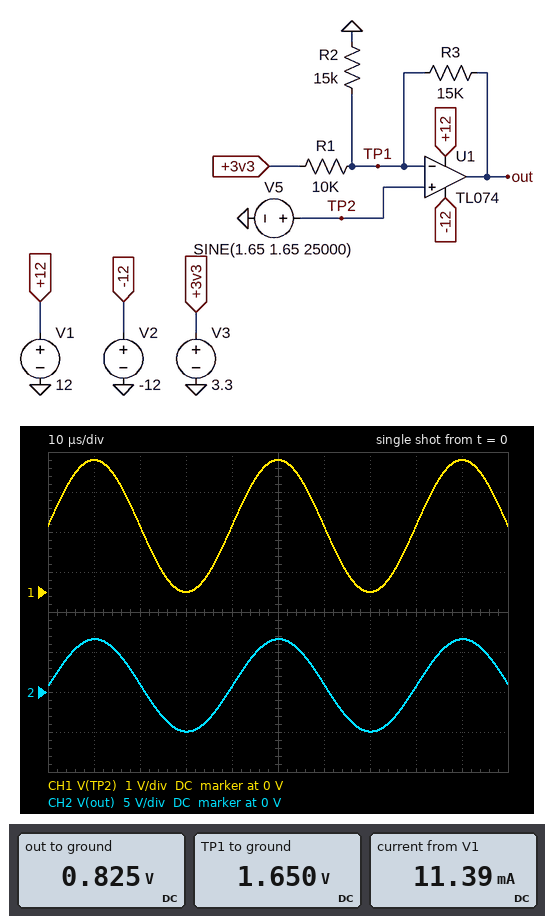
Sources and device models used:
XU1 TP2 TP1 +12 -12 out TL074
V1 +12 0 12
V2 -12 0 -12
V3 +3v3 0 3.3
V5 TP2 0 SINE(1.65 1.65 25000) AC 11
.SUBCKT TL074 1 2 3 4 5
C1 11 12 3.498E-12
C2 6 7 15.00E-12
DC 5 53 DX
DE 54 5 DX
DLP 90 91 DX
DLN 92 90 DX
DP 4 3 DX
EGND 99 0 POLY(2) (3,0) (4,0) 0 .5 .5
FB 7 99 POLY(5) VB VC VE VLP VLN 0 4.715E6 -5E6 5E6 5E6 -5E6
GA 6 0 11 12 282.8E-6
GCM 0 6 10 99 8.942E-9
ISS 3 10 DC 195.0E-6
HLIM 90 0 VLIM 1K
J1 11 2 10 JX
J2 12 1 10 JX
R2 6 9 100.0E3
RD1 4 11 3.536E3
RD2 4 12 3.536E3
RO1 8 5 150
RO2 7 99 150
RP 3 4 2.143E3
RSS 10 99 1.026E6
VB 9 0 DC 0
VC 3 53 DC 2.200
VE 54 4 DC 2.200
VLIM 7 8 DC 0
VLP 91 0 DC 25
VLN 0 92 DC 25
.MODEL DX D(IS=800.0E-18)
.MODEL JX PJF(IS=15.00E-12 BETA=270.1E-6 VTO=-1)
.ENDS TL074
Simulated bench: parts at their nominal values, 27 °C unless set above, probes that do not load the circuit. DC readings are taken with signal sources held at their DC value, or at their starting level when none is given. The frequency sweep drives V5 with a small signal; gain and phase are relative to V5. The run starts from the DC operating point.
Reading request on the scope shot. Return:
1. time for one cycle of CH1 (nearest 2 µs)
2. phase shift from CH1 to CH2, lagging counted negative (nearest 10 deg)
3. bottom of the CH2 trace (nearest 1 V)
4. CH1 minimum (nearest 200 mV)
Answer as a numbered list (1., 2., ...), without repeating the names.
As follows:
1. 40 µs
2. 0 deg
3. -5 V
4. 0 V
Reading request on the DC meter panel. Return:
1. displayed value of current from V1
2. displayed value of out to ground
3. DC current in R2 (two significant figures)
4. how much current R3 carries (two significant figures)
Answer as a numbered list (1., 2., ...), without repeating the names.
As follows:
1. 11.39 mA
2. 0.825 V
3. 110 µA
4. 55 µA
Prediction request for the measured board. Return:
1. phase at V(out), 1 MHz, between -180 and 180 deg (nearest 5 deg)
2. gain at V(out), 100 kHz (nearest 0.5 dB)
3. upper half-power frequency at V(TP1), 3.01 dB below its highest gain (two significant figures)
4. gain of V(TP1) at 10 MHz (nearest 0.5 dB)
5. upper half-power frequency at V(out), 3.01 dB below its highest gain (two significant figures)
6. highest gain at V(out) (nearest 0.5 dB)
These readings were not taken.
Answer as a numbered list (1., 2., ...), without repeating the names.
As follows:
1. -50 deg
2. 11.0 dB
3. 1.1 MHz
4. -25.0 dB
5. 1.1 MHz
6. 11.0 dB
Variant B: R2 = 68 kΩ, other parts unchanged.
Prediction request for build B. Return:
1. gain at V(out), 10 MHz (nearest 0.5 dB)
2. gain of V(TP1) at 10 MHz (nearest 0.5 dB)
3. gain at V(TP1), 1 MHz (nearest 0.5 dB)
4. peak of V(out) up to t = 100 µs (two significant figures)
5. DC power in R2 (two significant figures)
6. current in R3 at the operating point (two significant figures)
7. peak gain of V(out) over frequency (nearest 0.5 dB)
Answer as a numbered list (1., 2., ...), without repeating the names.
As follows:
1. -14.0 dB
2. -23.0 dB
3. -1.5 dB
4. 4.0 V
5. 40 µW
6. 140 µA
7. 8.5 dB
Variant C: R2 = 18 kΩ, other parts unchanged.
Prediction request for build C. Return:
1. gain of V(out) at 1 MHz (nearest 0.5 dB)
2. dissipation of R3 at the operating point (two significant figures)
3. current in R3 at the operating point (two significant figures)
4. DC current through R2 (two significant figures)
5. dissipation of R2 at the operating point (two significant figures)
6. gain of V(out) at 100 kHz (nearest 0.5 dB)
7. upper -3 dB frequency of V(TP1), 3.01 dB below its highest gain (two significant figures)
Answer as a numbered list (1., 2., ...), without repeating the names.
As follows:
1. 8.0 dB
2. 81 µW
3. 73 µA
4. 92 µA
5. 150 µW
6. 10.5 dB
7. 1.2 MHz
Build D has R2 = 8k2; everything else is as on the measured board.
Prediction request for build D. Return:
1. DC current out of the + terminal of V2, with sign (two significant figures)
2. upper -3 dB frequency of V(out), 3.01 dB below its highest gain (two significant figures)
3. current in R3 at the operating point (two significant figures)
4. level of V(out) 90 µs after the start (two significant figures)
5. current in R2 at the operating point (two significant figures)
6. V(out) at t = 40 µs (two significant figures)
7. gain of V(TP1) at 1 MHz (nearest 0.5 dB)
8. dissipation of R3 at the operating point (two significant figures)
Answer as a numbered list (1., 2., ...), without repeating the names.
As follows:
1. -11 mA
2. 890 kHz
3. 36 µA
4. 9.3 V
5. 200 µA
6. 2.0 V
7. -3.5 dB
8. 20 µW
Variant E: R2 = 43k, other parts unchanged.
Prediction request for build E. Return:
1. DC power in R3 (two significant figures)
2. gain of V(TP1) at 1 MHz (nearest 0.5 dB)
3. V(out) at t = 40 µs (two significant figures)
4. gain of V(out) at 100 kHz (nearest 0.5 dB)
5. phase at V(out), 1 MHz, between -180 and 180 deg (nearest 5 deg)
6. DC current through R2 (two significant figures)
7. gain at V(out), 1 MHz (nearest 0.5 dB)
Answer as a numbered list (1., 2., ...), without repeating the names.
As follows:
1. 240 µW
2. -1.5 dB
3. -350 mV
4. 9.0 dB
5. -45 deg
6. 38 µA
7. 7.5 dB
